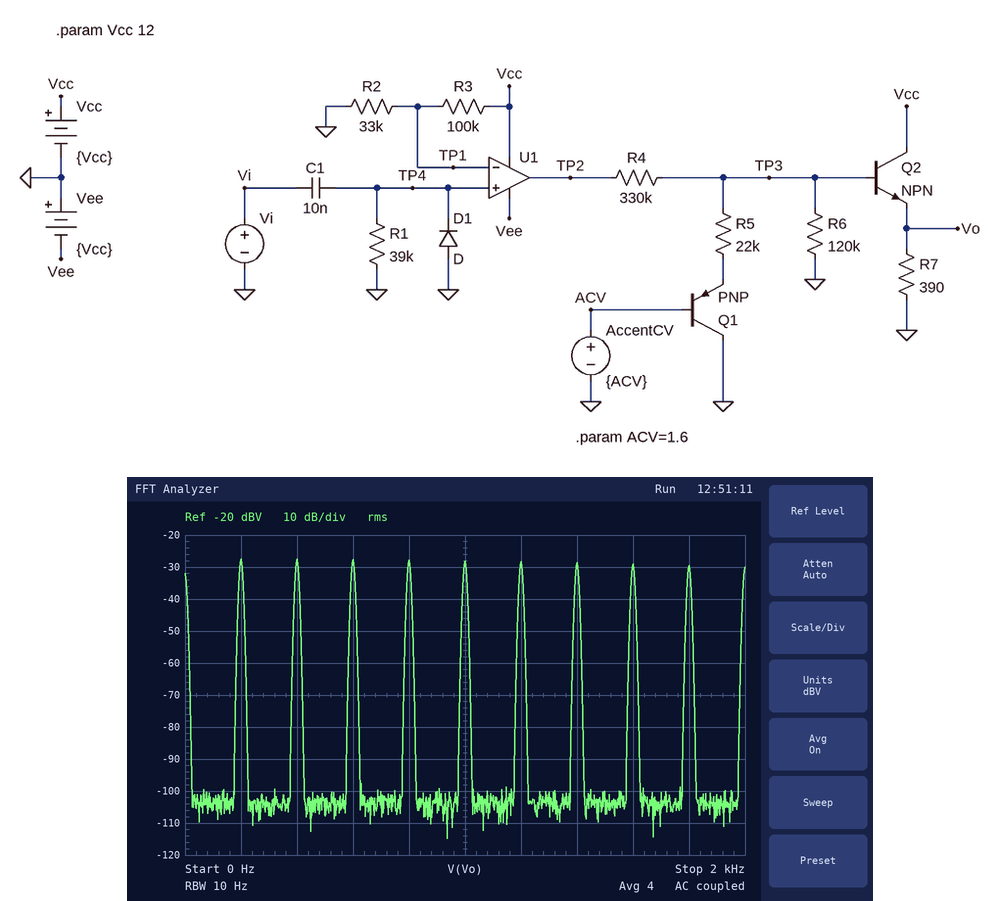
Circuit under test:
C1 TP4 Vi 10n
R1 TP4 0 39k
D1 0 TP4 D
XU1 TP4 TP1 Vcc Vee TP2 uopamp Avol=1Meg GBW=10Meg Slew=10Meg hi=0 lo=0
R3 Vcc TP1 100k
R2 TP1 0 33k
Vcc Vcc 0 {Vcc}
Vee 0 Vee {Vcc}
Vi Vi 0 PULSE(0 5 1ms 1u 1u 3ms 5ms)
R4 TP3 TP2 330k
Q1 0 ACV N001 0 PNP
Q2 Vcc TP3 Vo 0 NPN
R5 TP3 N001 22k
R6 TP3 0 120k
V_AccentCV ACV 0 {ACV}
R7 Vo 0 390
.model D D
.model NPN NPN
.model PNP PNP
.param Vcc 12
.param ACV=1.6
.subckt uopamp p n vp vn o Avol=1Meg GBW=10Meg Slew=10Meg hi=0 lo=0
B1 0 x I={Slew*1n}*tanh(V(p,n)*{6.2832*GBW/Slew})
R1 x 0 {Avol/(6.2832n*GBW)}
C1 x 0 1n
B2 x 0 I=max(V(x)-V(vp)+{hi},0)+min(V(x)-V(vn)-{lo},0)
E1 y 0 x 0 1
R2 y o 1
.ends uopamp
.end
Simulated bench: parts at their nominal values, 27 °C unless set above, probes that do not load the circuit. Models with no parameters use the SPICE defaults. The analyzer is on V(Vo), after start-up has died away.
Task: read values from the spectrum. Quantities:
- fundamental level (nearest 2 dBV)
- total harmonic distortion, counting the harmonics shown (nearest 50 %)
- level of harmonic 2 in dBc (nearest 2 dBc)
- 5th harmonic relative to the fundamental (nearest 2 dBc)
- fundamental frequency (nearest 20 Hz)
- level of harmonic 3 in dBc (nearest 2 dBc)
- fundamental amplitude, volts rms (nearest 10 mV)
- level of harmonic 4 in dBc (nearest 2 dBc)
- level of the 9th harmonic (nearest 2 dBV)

-28 dBV
250 %
0 dBc
0 dBc
200 Hz
0 dBc
40 mV
0 dBc
-30 dBV
